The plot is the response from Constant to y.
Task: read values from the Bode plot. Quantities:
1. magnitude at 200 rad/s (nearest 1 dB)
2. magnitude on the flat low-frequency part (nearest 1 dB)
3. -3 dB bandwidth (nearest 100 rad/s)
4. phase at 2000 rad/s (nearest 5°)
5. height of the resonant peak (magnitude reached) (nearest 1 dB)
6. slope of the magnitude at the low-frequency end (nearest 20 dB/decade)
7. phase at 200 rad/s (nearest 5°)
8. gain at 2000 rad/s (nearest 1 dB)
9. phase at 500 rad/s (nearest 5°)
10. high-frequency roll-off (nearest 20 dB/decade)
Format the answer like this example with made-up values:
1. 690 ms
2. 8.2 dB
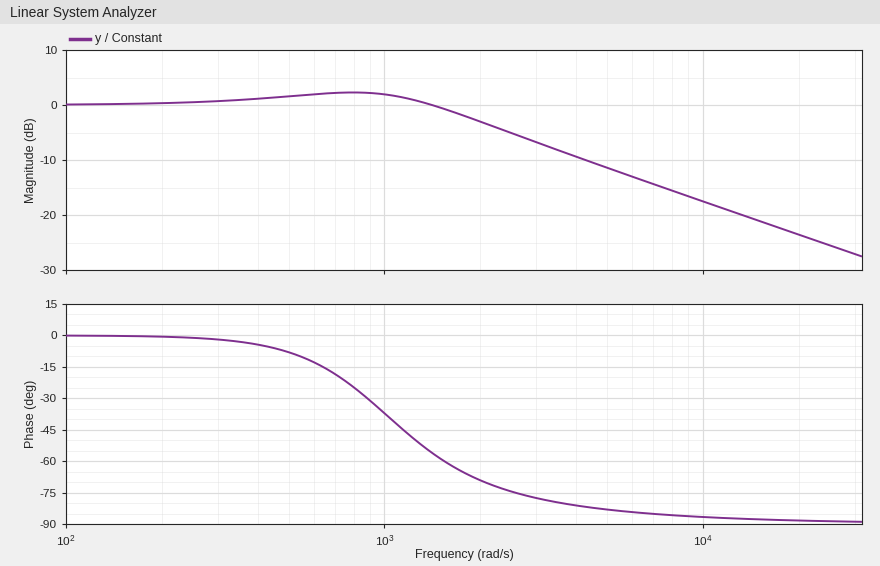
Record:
1. 0 dB
2. 0 dB
3. 2000 rad/s
4. -70°
5. 2 dB
6. 0 dB/decade
7. 0°
8. -3 dB
9. -10°
10. -20 dB/decade
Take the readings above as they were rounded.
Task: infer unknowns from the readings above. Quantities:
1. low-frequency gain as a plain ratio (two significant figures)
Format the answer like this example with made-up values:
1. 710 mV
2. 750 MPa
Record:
1. 1.0
